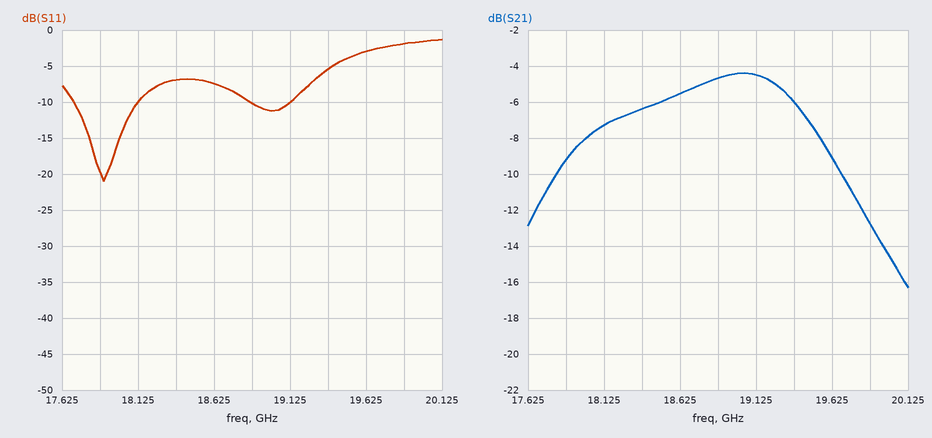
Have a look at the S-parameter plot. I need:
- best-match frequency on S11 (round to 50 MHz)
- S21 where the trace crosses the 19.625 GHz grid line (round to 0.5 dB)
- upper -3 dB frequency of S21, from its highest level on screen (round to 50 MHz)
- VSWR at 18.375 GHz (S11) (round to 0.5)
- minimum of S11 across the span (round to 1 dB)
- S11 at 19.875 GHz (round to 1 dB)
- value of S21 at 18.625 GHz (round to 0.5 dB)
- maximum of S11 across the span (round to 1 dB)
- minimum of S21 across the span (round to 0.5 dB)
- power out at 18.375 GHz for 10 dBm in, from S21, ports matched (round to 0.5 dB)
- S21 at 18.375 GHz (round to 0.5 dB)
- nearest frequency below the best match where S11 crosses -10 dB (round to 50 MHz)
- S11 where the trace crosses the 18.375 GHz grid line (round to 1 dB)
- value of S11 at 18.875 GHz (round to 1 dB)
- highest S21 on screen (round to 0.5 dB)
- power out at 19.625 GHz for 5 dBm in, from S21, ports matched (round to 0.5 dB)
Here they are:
17.90 GHz
-9.0 dB
19.50 GHz
2.5
-21 dB
-2 dB
-5.5 dB
-1 dB
-16.5 dB
3.5 dBm
-6.5 dB
17.70 GHz
-7 dB
-10 dB
-4.5 dB
-4.0 dBm
